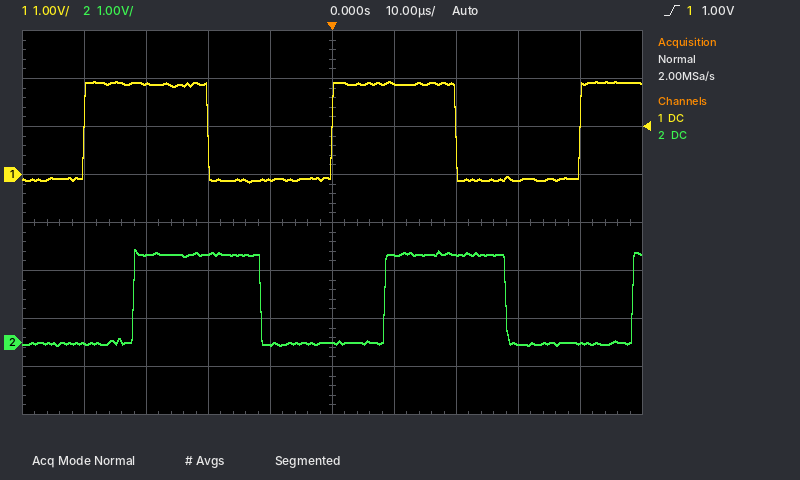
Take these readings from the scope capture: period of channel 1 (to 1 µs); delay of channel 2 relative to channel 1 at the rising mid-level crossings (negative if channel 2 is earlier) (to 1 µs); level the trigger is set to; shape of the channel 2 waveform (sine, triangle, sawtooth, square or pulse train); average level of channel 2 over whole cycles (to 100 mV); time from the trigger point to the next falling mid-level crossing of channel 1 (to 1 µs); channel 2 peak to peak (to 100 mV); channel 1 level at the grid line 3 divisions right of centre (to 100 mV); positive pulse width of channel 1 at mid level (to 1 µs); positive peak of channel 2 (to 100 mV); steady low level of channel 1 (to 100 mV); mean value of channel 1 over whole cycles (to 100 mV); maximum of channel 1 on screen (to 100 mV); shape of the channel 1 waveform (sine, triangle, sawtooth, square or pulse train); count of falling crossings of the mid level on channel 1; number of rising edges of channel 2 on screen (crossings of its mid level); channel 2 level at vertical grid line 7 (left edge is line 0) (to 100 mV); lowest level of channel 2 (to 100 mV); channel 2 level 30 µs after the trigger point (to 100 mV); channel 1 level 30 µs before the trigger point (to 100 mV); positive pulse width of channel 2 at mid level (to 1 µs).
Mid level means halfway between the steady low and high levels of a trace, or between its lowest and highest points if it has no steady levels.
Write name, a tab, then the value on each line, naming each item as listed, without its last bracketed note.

period of channel 1	40 µs
delay of channel 2 relative to channel 1 at the rising mid-level crossings (negative if channel 2 is earlier)	+8 µs
level the trigger is set to	1.00 V
shape of the channel 2 waveform	square
average level of channel 2 over whole cycles	900 mV
time from the trigger point to the next falling mid-level crossing of channel 1	20 µs
channel 2 peak to peak	2.0 V
channel 1 level at the grid line 3 divisions right of centre	-100 mV
positive pulse width of channel 1 at mid level	20 µs
positive peak of channel 2	1.9 V
steady low level of channel 1	-100 mV
mean value of channel 1 over whole cycles	900 mV
maximum of channel 1 on screen	1.9 V
shape of the channel 1 waveform	square
count of falling crossings of the mid level on channel 1	2
number of rising edges of channel 2 on screen	3
channel 2 level at vertical grid line 7 (left edge is line 0)	1.8 V
lowest level of channel 2	-100 mV
channel 2 level 30 µs after the trigger point	0.0 V
channel 1 level 30 µs before the trigger point	1.9 V
positive pulse width of channel 2 at mid level	20 µs
